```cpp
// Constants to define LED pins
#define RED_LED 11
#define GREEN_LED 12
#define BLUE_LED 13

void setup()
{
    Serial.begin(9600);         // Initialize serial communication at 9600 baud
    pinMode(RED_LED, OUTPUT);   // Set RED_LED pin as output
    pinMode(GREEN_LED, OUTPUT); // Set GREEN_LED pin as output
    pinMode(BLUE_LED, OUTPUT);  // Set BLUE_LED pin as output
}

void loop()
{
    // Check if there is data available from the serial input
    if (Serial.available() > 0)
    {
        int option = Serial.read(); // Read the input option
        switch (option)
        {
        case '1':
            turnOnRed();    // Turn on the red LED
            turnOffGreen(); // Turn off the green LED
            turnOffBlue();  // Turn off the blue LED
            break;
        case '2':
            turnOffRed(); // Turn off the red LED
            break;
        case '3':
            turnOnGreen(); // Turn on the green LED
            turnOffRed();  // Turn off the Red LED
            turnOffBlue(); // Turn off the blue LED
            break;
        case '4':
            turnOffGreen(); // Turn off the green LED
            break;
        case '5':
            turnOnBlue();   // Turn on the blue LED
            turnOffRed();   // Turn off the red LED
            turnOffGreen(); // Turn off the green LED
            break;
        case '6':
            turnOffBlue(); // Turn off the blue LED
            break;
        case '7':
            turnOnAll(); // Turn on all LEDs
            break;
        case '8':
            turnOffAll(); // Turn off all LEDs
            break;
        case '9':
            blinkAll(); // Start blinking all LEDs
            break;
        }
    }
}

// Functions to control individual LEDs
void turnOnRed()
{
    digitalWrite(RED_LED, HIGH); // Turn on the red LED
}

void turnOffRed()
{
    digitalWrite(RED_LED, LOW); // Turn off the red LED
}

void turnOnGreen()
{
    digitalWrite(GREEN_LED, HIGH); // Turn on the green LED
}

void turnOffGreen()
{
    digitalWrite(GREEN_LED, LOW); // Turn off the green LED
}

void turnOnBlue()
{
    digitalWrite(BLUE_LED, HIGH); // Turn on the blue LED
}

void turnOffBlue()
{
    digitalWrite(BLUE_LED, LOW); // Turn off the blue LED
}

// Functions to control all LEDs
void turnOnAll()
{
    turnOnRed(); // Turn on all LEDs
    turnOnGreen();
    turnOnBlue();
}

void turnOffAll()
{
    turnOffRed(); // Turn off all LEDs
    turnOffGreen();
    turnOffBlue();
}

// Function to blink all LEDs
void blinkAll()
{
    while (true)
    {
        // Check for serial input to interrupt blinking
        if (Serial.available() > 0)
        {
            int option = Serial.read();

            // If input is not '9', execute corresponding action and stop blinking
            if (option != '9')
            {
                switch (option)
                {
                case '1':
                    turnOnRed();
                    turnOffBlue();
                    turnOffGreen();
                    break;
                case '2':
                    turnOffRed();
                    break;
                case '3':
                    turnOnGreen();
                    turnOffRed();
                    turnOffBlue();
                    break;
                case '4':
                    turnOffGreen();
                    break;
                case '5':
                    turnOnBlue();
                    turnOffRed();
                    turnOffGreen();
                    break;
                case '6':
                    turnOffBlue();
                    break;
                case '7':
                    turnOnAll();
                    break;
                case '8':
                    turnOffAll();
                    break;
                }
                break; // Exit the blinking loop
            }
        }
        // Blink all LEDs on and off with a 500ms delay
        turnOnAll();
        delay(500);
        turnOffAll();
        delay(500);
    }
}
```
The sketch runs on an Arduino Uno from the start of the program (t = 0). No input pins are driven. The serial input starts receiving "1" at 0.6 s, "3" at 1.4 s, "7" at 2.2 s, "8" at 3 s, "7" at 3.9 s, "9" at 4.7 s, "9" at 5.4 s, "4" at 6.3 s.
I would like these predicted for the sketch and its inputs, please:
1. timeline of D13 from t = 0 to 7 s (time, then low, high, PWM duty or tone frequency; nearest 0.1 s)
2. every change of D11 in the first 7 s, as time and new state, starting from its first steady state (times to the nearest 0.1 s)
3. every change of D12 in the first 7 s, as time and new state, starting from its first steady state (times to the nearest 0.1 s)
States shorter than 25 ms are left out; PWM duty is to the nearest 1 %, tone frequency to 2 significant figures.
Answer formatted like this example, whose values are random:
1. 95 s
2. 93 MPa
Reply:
1. 0 s low; 2.2 s high; 3 s low; 3.9 s high; 5.2 s low; 5.7 s high; 6.2 s low
2. 0 s low; 0.6 s high; 1.4 s low; 2.2 s high; 3 s low; 3.9 s high; 5.2 s low; 5.7 s high; 6.2 s low
3. 0 s low; 1.4 s high; 3 s low; 3.9 s high; 5.2 s low; 5.7 s high; 6.2 s low
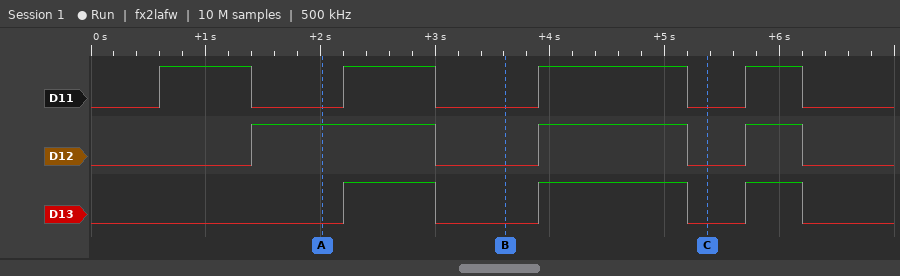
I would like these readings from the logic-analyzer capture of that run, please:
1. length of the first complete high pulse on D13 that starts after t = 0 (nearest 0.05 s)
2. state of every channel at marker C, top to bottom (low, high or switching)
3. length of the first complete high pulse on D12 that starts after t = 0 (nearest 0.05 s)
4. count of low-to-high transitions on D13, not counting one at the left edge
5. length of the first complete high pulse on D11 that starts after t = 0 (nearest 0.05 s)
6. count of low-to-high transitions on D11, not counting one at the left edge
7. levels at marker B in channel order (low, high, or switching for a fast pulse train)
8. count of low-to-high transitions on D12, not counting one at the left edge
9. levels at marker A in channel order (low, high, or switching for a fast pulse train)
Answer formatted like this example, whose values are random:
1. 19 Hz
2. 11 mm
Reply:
1. 0.80 s
2. D11 low, D12 low, D13 low
3. 1.60 s
4. 3
5. 0.80 s
6. 4
7. D11 low, D12 low, D13 low
8. 3
9. D11 low, D12 high, D13 low
